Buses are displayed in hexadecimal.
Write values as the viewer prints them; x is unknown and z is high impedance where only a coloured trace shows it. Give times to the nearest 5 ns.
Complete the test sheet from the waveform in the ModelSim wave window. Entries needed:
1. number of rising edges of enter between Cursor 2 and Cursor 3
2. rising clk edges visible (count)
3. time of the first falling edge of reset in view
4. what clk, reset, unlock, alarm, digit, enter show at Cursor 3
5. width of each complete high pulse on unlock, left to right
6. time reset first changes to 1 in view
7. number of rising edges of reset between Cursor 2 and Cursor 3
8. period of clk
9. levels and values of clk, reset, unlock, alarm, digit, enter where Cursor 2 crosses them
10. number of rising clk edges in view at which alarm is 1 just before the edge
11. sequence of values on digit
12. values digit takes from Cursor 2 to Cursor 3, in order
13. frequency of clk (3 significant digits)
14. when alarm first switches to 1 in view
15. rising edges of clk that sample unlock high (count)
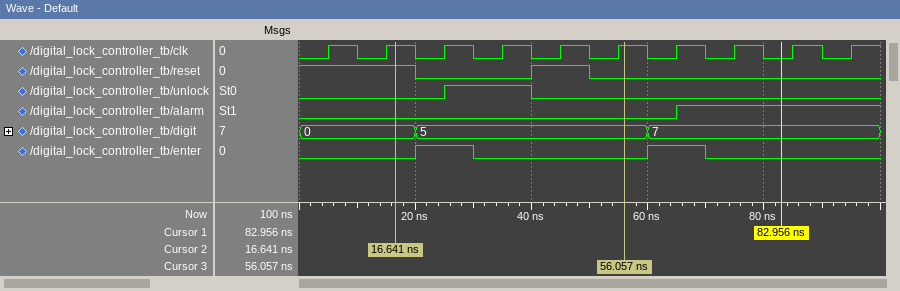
1
10
20 ns
clk=1, reset=0, unlock=0, alarm=0, digit=5, enter=0
15 ns
40 ns
1
10 ns
clk=1, reset=1, unlock=0, alarm=0, digit=0, enter=0
3
0, 5, 7
0, 5
100 MHz
65 ns
1
